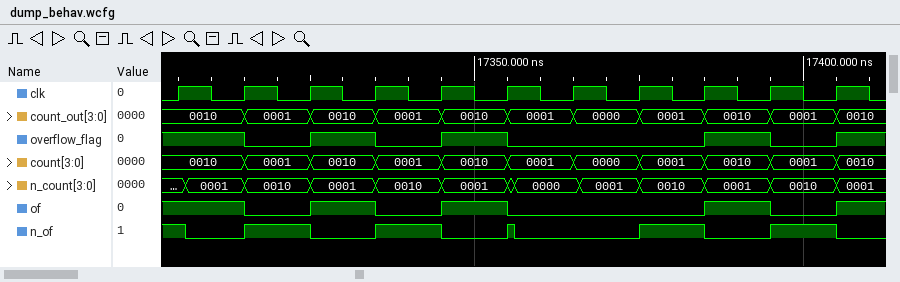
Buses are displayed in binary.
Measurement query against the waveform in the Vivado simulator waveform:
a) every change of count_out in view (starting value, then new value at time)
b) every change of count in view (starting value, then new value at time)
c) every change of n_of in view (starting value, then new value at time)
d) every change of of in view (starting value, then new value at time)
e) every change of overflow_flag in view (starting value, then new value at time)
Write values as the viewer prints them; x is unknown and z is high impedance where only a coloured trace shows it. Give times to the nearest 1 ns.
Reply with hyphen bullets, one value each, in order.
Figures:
- 0010, 0001 at 17315 ns, 0010 at 17325 ns, 0001 at 17335 ns, 0010 at 17345 ns, 0001 at 17355 ns, 0000 at 17365 ns, 0001 at 17375 ns, 0010 at 17385 ns, 0001 at 17395 ns, 0010 at 17405 ns
- 0010, 0001 at 17315 ns, 0010 at 17325 ns, 0001 at 17335 ns, 0010 at 17345 ns, 0001 at 17355 ns, 0000 at 17365 ns, 0001 at 17375 ns, 0010 at 17385 ns, 0001 at 17395 ns, 0010 at 17405 ns
- 1, 0 at 17306 ns, 1 at 17315 ns, 0 at 17325 ns, 1 at 17335 ns, 0 at 17345 ns, 1 at 17355 ns, 0 at 17356 ns, 1 at 17375 ns, 0 at 17385 ns, 1 at 17395 ns, 0 at 17405 ns
- 1, 0 at 17315 ns, 1 at 17325 ns, 0 at 17335 ns, 1 at 17345 ns, 0 at 17355 ns, 1 at 17385 ns, 0 at 17395 ns, 1 at 17405 ns
- 1, 0 at 17315 ns, 1 at 17325 ns, 0 at 17335 ns, 1 at 17345 ns, 0 at 17355 ns, 1 at 17385 ns, 0 at 17395 ns, 1 at 17405 ns
